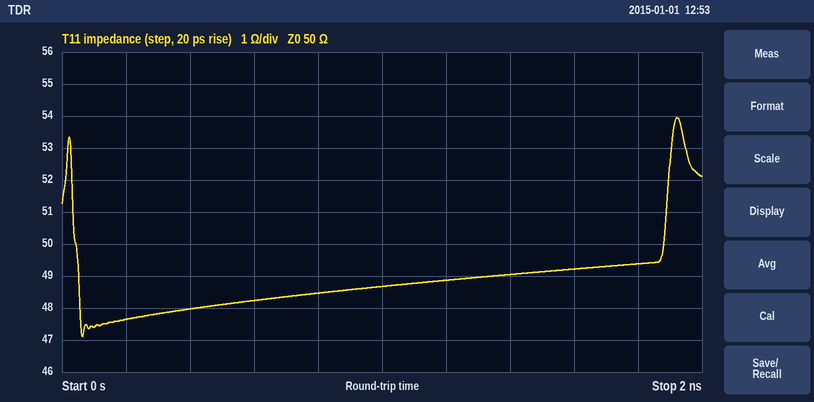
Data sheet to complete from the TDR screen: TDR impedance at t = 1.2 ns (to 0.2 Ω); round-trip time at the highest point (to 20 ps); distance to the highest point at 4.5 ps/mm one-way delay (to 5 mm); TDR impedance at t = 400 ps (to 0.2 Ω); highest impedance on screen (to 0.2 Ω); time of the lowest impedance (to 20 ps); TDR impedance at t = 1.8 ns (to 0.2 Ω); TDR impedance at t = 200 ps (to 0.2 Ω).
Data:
48.8 Ω
1.92 ns
215 mm
48.0 Ω
54.0 Ω
60 ps
49.4 Ω
47.6 Ω
